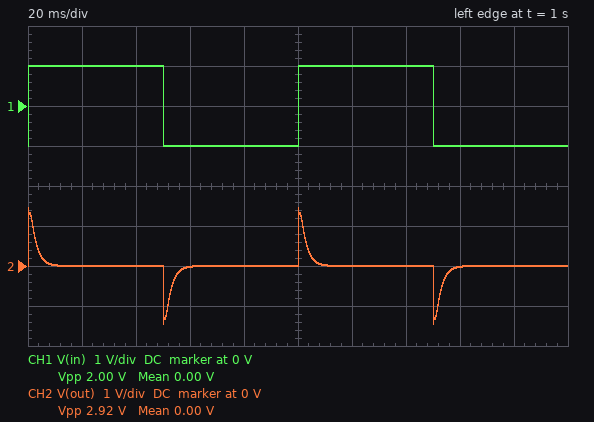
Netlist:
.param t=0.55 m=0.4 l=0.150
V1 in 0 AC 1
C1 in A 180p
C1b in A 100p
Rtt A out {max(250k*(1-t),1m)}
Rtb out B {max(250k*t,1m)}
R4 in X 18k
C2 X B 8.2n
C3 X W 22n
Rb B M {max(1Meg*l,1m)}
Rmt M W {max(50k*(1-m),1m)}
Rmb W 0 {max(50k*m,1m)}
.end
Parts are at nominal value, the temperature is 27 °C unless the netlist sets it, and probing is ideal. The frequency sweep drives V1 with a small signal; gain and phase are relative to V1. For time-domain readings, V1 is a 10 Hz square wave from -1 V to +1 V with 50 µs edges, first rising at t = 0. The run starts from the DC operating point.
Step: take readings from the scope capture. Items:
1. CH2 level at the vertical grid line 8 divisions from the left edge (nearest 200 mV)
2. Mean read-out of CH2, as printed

0 V
0.00 V
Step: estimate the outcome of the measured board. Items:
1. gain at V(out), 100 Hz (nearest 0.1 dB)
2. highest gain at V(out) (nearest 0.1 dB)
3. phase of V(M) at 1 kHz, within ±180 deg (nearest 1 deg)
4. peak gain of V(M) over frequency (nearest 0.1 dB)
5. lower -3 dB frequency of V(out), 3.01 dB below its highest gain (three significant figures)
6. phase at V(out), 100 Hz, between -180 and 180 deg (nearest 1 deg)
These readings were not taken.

-2.0 dB
-1.5 dB
8 deg
-5.3 dB
54.1 Hz
28 deg
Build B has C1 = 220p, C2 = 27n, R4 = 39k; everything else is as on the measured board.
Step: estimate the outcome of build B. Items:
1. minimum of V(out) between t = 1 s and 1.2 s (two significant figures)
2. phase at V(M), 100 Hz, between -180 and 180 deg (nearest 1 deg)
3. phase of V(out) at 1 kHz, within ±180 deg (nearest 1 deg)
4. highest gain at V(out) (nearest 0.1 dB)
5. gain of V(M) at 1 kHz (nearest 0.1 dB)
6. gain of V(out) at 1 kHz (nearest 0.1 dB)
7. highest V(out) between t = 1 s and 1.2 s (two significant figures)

-1.3 V
20 deg
11 deg
-2.3 dB
-9.3 dB
-7.3 dB
1.3 V
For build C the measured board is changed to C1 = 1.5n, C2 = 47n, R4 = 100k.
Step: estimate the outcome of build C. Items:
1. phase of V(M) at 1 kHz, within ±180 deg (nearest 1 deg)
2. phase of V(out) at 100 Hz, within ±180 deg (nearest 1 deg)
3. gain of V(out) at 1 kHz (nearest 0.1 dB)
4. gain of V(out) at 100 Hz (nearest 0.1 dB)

5 deg
-11 deg
-4.5 dB
-6.5 dB
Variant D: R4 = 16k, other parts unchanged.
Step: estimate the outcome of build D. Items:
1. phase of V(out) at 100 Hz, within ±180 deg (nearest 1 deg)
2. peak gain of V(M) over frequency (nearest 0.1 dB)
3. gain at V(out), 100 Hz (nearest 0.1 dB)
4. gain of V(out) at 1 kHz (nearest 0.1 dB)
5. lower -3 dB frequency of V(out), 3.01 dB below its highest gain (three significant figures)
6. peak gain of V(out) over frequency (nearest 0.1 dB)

29 deg
-4.9 dB
-1.9 dB
-4.0 dB
55.6 Hz
-1.3 dB
